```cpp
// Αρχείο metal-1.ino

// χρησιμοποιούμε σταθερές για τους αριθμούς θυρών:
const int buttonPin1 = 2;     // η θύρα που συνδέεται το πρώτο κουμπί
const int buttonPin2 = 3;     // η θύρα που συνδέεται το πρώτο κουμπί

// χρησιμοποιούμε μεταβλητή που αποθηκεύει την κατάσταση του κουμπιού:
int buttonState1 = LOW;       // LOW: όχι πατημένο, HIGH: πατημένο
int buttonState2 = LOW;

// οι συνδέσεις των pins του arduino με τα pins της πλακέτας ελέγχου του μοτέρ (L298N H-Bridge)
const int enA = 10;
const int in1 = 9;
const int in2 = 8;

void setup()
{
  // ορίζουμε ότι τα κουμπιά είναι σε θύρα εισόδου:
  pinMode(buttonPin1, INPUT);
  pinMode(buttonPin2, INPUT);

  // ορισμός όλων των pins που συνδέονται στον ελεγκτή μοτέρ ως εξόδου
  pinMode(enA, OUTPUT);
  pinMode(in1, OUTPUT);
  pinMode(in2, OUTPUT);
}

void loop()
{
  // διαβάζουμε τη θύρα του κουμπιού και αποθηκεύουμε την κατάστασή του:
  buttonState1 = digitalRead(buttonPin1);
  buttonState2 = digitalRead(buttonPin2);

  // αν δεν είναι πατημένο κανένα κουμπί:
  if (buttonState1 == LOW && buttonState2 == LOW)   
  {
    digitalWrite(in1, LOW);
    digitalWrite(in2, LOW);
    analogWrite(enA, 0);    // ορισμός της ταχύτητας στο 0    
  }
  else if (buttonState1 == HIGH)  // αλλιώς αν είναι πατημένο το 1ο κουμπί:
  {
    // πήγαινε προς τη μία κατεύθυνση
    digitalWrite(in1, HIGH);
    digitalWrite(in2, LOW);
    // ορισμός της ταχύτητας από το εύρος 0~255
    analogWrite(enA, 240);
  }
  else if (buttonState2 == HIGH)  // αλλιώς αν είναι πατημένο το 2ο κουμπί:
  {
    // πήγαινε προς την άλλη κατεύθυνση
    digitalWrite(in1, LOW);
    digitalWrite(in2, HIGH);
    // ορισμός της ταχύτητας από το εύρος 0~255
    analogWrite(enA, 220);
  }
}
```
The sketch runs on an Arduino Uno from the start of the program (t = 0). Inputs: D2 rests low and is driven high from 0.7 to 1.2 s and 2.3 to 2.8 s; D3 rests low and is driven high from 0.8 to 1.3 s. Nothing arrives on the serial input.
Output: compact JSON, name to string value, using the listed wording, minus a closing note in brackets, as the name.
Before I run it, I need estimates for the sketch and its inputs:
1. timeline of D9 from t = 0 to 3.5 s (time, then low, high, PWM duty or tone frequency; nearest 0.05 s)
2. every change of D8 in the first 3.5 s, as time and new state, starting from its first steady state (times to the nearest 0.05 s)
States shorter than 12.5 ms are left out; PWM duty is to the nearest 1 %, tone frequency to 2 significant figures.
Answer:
{"timeline of D9 from t = 0 to 3.5 s": "0 s low; 0.7 s high; 1.2 s low; 2.3 s high; 2.8 s low", "every change of D8 in the first 3.5 s, as time and new state, starting from its first steady state": "0 s low; 1.2 s high; 1.3 s low"}
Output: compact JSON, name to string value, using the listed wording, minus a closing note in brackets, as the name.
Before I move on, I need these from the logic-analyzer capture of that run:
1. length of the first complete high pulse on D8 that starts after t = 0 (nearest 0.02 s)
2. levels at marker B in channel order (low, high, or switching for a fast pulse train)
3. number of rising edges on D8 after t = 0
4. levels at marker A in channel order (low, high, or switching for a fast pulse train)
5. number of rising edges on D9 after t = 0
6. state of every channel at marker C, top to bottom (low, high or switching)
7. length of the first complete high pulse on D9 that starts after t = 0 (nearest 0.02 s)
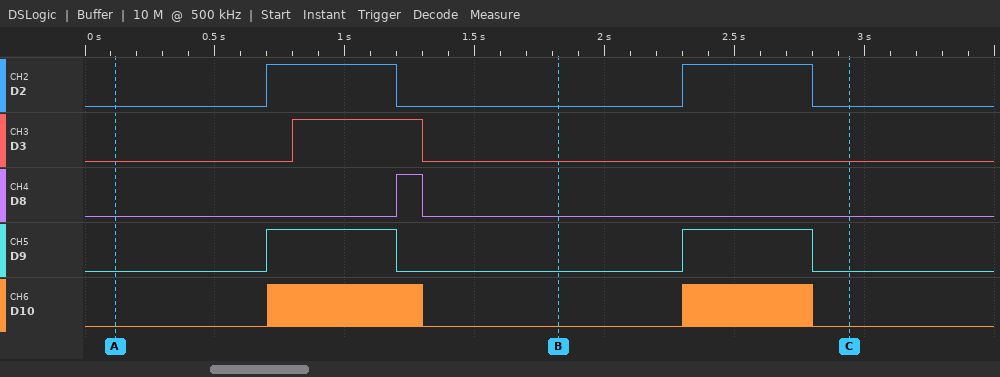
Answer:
{"length of the first complete high pulse on D8 that starts after t = 0": "0.10 s", "levels at marker B in channel order": "D2 low, D3 low, D8 low, D9 low, D10 low", "number of rising edges on D8 after t = 0": "1", "levels at marker A in channel order": "D2 low, D3 low, D8 low, D9 low, D10 low", "number of rising edges on D9 after t = 0": "2", "state of every channel at marker C, top to bottom": "D2 low, D3 low, D8 low, D9 low, D10 low", "length of the first complete high pulse on D9 that starts after t = 0": "0.50 s"}
